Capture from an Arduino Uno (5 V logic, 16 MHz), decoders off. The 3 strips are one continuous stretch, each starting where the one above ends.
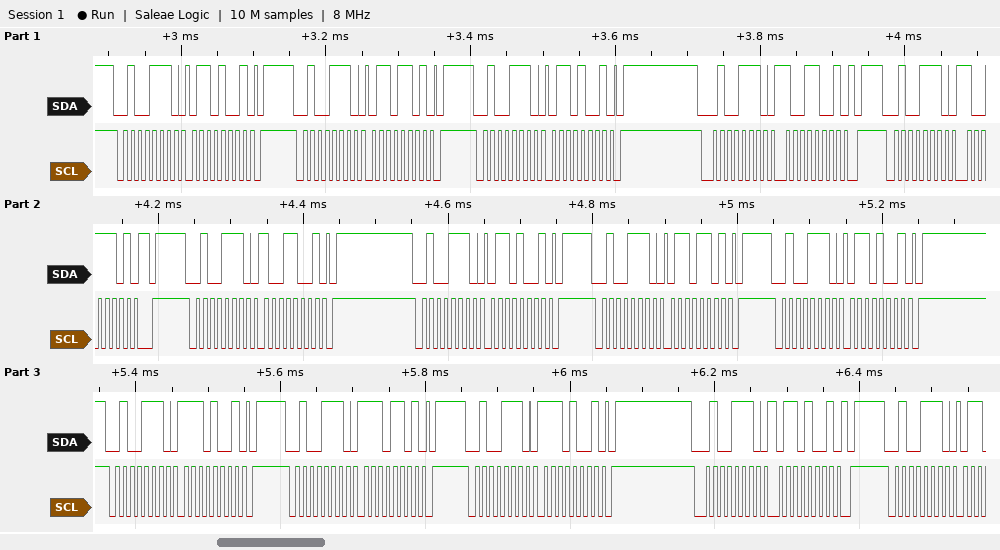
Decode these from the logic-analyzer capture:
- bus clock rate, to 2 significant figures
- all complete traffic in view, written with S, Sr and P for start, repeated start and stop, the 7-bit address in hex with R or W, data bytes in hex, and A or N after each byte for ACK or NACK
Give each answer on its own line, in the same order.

100 kHz
S 27W A 69 A P S 27W A 6D A P S 27W A 69 A P S 27W A 99 A P S 27W A 9D A P S 27W A 99 A P S 27W A 69 A P S 27W A 6D A P S 27W A 69 A P S 27W A E9 A P S 27W A ED A P S 27W A E9 A P S 27W A 69 A P S 27W A
